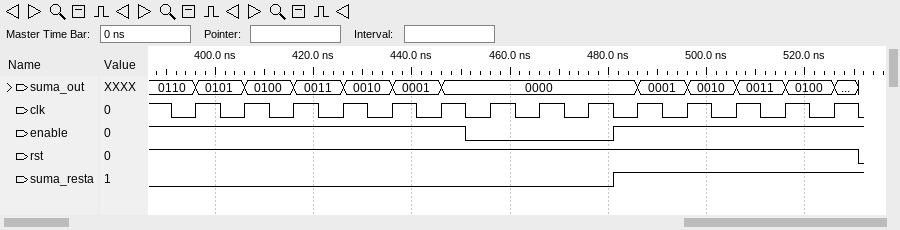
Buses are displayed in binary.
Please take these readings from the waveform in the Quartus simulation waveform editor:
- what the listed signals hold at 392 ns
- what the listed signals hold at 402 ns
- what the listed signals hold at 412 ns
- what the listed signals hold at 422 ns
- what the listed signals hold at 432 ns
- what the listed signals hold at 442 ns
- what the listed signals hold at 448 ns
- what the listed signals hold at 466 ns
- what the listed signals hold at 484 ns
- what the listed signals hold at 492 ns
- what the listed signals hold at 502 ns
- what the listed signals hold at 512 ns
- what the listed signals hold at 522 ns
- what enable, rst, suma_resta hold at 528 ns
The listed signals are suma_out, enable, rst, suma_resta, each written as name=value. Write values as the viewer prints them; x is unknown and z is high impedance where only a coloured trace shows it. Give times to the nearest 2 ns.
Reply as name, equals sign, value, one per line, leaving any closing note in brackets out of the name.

what the listed signals hold at 392 ns = suma_out=0110, enable=1, rst=1, suma_resta=0
what the listed signals hold at 402 ns = suma_out=0101, enable=1, rst=1, suma_resta=0
what the listed signals hold at 412 ns = suma_out=0100, enable=1, rst=1, suma_resta=0
what the listed signals hold at 422 ns = suma_out=0011, enable=1, rst=1, suma_resta=0
what the listed signals hold at 432 ns = suma_out=0010, enable=1, rst=1, suma_resta=0
what the listed signals hold at 442 ns = suma_out=0001, enable=1, rst=1, suma_resta=0
what the listed signals hold at 448 ns = suma_out=0000, enable=1, rst=1, suma_resta=0
what the listed signals hold at 466 ns = suma_out=0000, enable=0, rst=1, suma_resta=0
what the listed signals hold at 484 ns = suma_out=0000, enable=1, rst=1, suma_resta=1
what the listed signals hold at 492 ns = suma_out=0001, enable=1, rst=1, suma_resta=1
what the listed signals hold at 502 ns = suma_out=0010, enable=1, rst=1, suma_resta=1
what the listed signals hold at 512 ns = suma_out=0011, enable=1, rst=1, suma_resta=1
what the listed signals hold at 522 ns = suma_out=0100, enable=1, rst=1, suma_resta=1
what enable, rst, suma_resta hold at 528 ns = enable=1, rst=1, suma_resta=1
